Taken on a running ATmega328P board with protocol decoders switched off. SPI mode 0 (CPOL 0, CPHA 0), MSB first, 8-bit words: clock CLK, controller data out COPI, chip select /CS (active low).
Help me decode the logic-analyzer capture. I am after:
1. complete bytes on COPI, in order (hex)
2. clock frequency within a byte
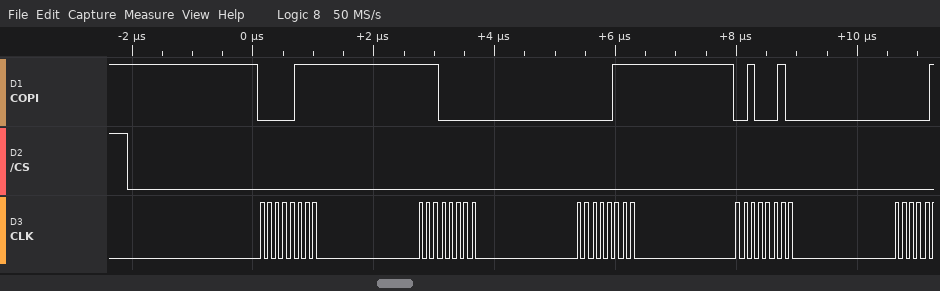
0x07 0xE0 0x07 0x22
8 MHz
